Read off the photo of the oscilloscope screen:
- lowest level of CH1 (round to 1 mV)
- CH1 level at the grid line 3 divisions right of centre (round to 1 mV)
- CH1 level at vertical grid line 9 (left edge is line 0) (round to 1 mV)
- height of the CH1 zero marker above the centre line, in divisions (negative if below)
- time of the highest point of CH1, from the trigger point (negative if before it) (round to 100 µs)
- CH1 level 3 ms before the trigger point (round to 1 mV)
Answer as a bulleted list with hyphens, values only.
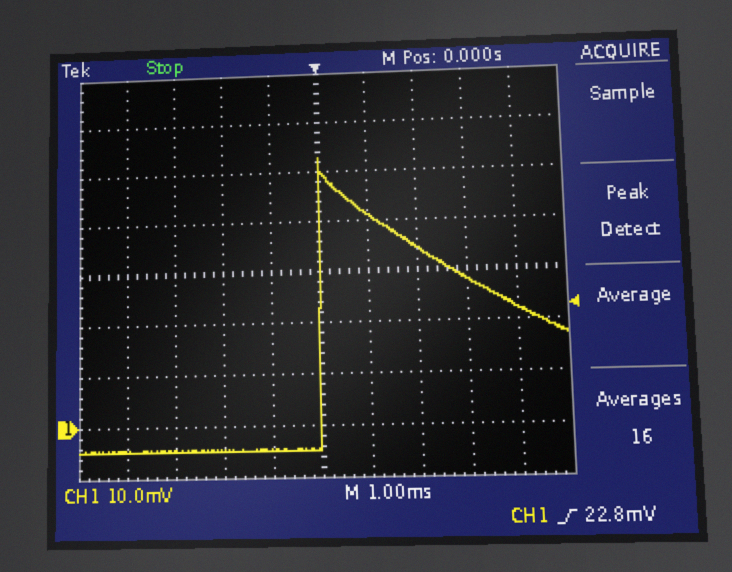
- -5 mV
- 28 mV
- 22 mV
- -3.0 div
- 0.0 ms
- -5 mV
